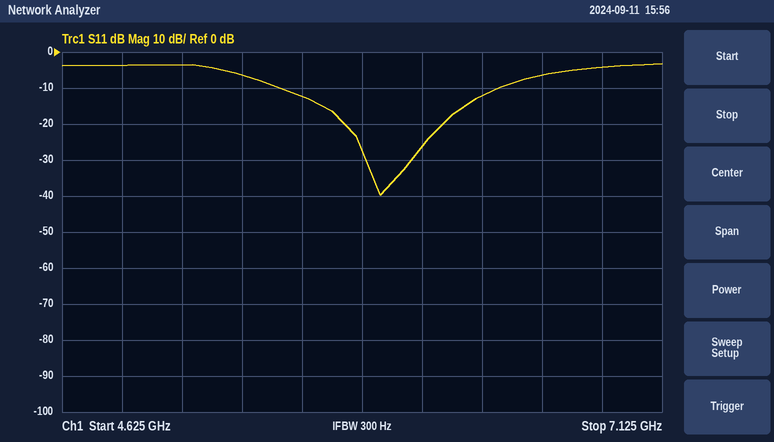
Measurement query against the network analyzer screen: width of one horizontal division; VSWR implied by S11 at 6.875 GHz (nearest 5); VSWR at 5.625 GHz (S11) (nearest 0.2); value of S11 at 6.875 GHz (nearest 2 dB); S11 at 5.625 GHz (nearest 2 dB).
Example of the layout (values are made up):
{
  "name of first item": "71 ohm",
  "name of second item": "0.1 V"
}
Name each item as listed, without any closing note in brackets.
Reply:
{
  "width of one horizontal division": "250 MHz",
  "VSWR implied by S11 at 6.875 GHz": "5",
  "VSWR at 5.625 GHz (S11)": "1.6",
  "value of S11 at 6.875 GHz": "-4 dB",
  "S11 at 5.625 GHz": "-12 dB"
}
